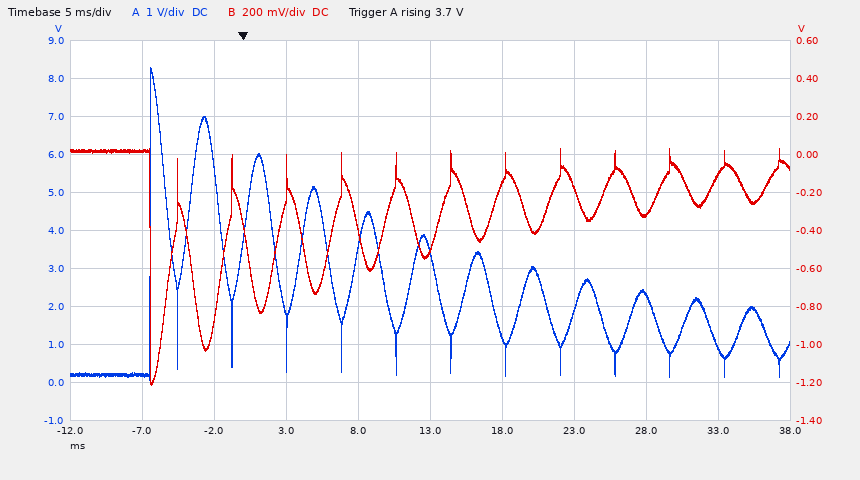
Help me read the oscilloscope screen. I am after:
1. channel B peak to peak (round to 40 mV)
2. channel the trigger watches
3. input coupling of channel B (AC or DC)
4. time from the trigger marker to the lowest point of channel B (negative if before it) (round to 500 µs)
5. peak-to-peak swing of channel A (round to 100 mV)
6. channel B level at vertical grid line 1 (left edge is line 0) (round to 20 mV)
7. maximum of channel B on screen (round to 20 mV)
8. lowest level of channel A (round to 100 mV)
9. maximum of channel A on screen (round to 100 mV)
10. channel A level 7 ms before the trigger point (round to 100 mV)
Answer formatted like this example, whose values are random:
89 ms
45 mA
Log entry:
1.24 V
channel A
DC
-6.5 ms
8.2 V
20 mV
40 mV
100 mV
8.3 V
200 mV
